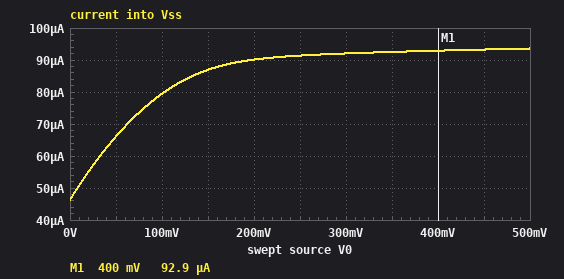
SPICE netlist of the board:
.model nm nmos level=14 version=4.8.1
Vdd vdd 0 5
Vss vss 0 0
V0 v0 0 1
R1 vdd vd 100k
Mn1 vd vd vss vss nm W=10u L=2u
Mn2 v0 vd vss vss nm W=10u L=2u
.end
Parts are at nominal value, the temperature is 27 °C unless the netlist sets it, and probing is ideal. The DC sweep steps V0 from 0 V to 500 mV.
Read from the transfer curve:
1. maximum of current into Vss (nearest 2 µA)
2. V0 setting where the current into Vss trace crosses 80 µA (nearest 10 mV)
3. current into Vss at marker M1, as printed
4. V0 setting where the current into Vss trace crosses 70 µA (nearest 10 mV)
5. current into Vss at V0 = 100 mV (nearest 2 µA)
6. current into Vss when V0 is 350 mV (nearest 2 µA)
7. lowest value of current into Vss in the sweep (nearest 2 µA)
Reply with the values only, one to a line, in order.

94 µA
100 mV
92.9 µA
60 mV
80 µA
92 µA
46 µA
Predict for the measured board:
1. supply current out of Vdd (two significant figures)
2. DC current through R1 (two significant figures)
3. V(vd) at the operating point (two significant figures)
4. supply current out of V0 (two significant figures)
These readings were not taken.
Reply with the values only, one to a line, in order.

46 µA
46 µA
370 mV
50 µA
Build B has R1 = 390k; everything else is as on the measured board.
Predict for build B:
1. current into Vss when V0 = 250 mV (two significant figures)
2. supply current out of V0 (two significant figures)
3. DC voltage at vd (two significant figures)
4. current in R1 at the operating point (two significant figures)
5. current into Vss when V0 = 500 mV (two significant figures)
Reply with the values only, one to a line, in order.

24 µA
14 µA
280 mV
12 µA
25 µA
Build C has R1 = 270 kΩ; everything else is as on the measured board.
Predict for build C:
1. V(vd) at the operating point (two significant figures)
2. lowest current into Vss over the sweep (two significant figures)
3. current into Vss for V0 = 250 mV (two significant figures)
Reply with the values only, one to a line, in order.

300 mV
17 µA
35 µA
